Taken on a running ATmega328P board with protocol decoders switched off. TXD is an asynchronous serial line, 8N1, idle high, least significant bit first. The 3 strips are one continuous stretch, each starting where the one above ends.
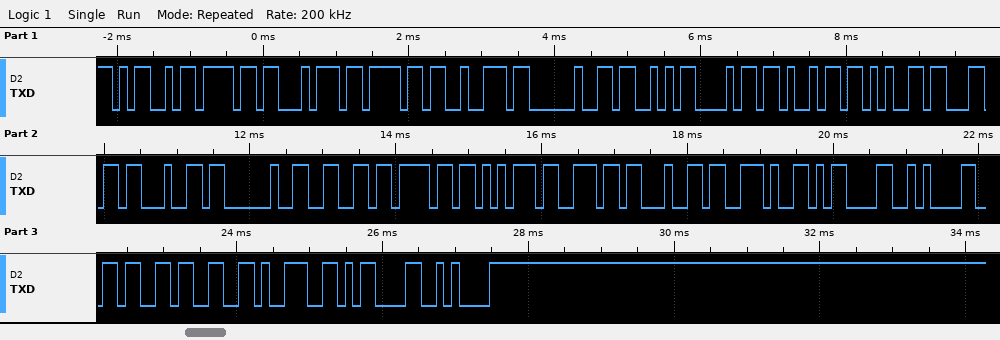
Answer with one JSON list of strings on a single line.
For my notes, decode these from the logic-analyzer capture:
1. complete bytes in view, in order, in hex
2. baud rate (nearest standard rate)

["4D 6F 74 6F 72 20 53 68 69 65 6C 64 20 66 6F 75 6E 64 2E 0D 0A 36 33 39 0D 0A", "9600 baud"]
